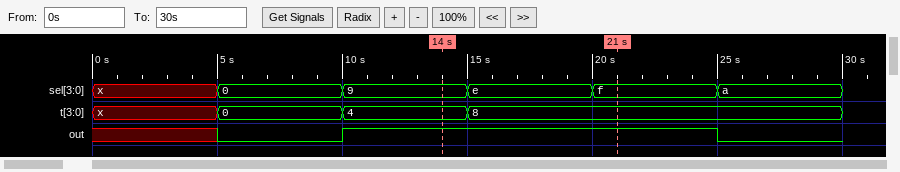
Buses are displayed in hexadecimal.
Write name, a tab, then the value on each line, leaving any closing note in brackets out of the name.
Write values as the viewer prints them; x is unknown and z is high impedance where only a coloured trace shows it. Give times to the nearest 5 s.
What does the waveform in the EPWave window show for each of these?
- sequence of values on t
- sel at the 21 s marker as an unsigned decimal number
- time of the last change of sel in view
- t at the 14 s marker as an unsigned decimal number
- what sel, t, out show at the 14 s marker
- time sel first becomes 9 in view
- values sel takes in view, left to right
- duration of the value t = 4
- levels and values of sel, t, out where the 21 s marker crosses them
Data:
sequence of values on t	x, 0, 4, 8
sel at the 21 s marker as an unsigned decimal number	15
time of the last change of sel in view	25 s
t at the 14 s marker as an unsigned decimal number	4
what sel, t, out show at the 14 s marker	sel=9, t=4, out=1
time sel first becomes 9 in view	10 s
values sel takes in view, left to right	x, 0, 9, e, f, a
duration of the value t = 4	5 s
levels and values of sel, t, out where the 21 s marker crosses them	sel=f, t=8, out=1
